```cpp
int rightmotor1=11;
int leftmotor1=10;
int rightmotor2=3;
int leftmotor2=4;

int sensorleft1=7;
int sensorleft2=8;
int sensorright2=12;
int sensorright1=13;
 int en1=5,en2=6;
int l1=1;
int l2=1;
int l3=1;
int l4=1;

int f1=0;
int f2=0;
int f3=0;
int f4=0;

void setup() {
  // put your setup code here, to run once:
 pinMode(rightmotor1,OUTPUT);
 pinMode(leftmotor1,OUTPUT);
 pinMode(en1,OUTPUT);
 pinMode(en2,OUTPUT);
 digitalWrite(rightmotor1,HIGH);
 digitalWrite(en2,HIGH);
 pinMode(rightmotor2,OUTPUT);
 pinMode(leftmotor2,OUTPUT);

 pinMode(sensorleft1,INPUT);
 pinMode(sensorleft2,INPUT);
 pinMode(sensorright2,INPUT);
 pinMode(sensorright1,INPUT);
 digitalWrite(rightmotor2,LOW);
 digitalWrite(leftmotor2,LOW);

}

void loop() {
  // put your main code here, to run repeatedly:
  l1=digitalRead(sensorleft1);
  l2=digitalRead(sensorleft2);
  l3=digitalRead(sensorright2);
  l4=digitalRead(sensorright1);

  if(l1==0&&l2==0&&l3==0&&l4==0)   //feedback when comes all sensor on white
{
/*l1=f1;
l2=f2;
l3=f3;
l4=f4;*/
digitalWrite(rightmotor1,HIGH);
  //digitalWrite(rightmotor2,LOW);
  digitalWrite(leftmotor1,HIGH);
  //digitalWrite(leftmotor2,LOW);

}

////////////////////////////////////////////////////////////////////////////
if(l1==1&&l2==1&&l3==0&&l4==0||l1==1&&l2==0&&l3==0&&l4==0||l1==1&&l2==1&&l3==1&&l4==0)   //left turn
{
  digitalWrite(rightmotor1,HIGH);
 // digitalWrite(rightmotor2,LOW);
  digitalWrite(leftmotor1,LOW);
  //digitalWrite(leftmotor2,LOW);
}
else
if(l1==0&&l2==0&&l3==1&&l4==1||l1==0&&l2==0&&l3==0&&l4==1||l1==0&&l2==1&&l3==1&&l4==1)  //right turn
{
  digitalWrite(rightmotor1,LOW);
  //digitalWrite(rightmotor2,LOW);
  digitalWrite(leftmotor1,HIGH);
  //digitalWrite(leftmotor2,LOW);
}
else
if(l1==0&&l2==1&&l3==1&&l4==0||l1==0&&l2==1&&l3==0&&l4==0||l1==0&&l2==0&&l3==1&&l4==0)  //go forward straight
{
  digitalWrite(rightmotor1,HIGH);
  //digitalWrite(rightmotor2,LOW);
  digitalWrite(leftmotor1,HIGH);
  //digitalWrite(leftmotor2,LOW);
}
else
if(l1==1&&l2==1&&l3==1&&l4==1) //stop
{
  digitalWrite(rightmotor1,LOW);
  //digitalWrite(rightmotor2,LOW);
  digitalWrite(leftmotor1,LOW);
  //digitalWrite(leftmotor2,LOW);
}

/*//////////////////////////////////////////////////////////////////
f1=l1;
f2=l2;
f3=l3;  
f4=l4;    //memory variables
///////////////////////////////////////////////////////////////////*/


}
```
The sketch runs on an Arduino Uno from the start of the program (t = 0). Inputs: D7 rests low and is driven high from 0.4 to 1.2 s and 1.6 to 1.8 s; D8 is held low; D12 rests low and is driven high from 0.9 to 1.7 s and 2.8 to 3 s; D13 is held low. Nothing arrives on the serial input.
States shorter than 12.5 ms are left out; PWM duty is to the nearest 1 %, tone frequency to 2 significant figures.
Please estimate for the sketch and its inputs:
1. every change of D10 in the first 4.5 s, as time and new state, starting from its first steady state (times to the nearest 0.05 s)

0 s high; 0.4 s low; 1.2 s high; 1.7 s low; 1.8 s high
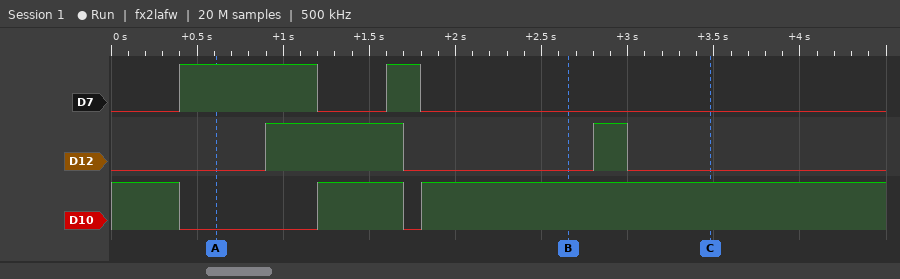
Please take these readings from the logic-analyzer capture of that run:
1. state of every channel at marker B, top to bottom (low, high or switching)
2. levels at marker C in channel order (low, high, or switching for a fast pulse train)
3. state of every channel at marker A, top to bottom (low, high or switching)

D7 low, D12 low, D10 high
D7 low, D12 low, D10 high
D7 high, D12 low, D10 low
